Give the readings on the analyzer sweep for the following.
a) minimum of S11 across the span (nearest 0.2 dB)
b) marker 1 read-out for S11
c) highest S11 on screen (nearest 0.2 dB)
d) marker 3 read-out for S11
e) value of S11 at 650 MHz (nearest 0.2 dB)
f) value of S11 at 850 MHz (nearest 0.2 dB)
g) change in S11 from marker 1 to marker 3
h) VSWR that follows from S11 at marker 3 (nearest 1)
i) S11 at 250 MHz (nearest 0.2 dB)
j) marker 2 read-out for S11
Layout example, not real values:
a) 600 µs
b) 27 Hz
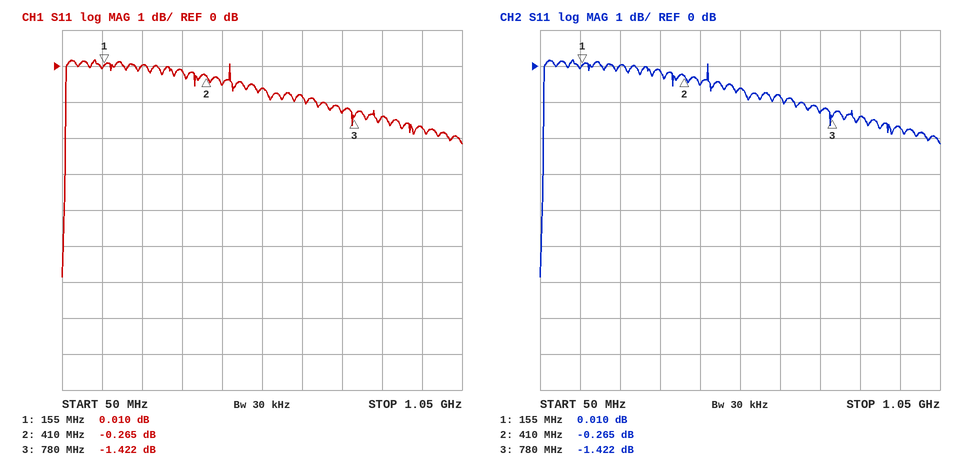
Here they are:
a) -5.8 dB
b) 0.010 dB
c) 0.2 dB
d) -1.422 dB
e) -0.8 dB
f) -1.4 dB
g) -1.432 dB
h) 12
i) 0.0 dB
j) -0.265 dB
